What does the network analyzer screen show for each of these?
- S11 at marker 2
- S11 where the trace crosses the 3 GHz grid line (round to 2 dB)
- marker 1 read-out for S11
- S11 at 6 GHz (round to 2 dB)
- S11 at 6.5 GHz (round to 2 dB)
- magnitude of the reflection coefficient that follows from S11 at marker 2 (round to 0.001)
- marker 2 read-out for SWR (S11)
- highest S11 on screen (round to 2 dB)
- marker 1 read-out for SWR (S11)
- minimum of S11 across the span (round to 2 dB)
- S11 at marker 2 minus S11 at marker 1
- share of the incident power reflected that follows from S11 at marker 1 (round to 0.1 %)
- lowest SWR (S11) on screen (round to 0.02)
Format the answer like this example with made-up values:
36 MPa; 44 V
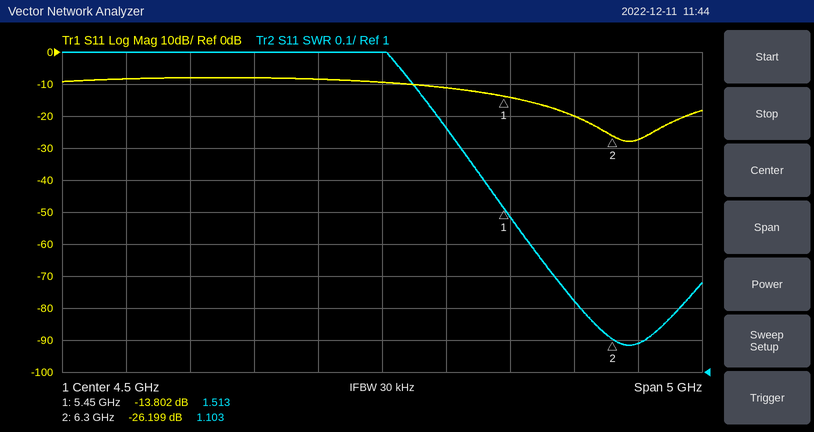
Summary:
-26.199 dB; -8 dB; -13.802 dB; -20 dB; -28 dB; 0.049; 1.103; -8 dB; 1.513; -28 dB; -12.397 dB; 4.2 %; 1.08
